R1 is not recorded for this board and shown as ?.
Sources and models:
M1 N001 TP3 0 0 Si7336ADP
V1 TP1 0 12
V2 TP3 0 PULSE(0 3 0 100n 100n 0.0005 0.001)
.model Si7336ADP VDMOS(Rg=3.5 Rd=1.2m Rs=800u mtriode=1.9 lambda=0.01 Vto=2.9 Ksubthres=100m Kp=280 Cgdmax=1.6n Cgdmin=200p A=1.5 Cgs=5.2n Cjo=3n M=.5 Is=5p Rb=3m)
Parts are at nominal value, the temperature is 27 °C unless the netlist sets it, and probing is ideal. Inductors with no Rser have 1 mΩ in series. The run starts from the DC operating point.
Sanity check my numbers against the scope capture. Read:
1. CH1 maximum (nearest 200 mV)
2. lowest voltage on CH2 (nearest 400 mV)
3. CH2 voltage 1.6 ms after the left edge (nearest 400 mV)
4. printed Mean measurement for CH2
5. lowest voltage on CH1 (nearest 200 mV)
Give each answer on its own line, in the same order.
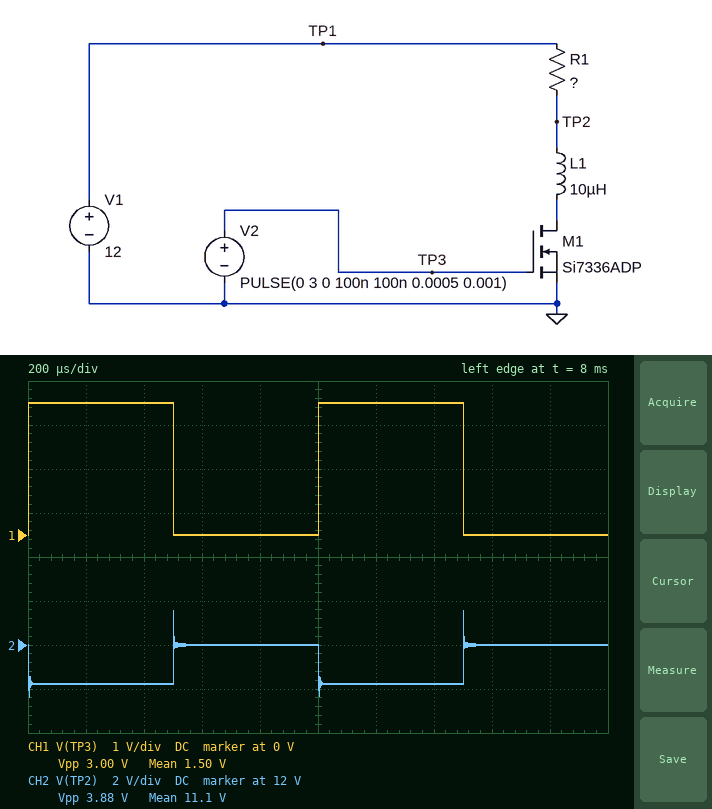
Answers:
3.0 V
9.6 V
12.0 V
11.1 V
0 V
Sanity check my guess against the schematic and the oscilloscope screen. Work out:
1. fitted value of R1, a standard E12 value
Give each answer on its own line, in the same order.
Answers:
0.68 Ω
